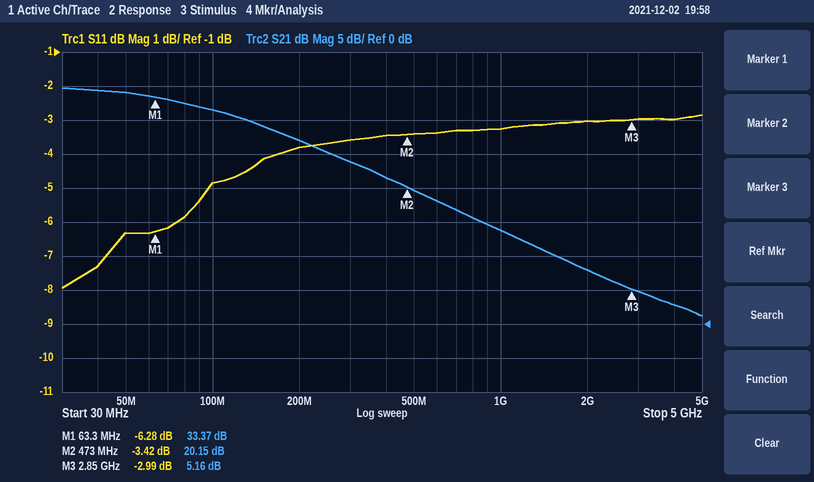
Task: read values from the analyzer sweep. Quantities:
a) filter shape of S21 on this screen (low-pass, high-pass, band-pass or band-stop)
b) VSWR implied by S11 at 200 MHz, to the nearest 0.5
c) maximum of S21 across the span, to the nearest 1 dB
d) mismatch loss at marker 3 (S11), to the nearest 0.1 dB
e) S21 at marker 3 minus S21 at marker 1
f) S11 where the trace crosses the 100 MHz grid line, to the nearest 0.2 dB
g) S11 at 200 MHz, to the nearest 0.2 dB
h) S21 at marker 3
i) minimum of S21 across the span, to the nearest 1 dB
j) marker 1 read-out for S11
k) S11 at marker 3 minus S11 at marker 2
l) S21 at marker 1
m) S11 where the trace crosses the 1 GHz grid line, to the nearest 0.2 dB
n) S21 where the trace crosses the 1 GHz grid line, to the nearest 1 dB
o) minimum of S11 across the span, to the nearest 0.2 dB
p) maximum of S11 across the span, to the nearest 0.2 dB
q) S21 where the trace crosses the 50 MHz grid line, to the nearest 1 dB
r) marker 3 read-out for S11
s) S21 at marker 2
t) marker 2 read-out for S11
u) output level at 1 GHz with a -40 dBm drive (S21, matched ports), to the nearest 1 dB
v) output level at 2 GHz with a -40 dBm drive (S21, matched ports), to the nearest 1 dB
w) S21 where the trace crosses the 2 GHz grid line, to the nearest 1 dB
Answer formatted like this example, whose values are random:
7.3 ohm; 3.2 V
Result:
low-pass; 4.5; 35 dB; 3.0 dB; -28.21 dB; -4.8 dB; -3.8 dB; 5.16 dB; 1 dB; -6.28 dB; 0.43 dB; 33.37 dB; -3.2 dB; 14 dB; -8.0 dB; -2.8 dB; 34 dB; -2.99 dB; 20.15 dB; -3.42 dB; -26 dBm; -32 dBm; 8 dB
